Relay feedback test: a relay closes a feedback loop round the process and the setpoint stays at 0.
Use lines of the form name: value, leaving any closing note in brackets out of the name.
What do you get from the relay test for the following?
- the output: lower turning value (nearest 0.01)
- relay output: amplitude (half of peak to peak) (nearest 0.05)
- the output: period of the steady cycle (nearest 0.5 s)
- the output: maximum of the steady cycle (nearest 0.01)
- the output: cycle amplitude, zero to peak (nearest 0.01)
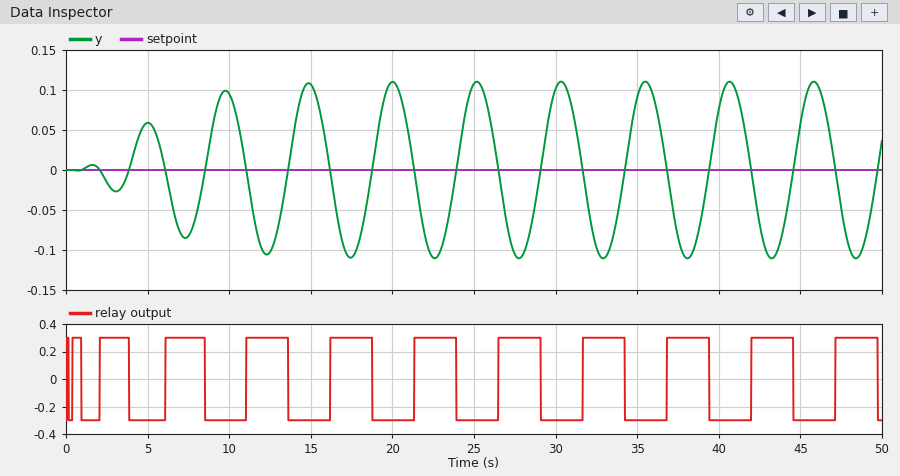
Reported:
the output: lower turning value: -0.11
relay output: amplitude (half of peak to peak): 0.30
the output: period of the steady cycle: 5.0 s
the output: maximum of the steady cycle: 0.11
the output: cycle amplitude, zero to peak: 0.11
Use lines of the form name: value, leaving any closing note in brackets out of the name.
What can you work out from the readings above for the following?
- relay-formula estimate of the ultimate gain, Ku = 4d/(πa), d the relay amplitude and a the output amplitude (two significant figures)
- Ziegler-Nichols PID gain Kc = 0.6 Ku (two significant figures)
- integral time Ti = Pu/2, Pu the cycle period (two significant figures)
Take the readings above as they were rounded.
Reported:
relay-formula estimate of the ultimate gain, Ku = 4d/(πa), d the relay amplitude and a the output amplitude: 3.5
Ziegler-Nichols PID gain Kc = 0.6 Ku: 2.1
integral time Ti = Pu/2, Pu the cycle period: 2.5 s
